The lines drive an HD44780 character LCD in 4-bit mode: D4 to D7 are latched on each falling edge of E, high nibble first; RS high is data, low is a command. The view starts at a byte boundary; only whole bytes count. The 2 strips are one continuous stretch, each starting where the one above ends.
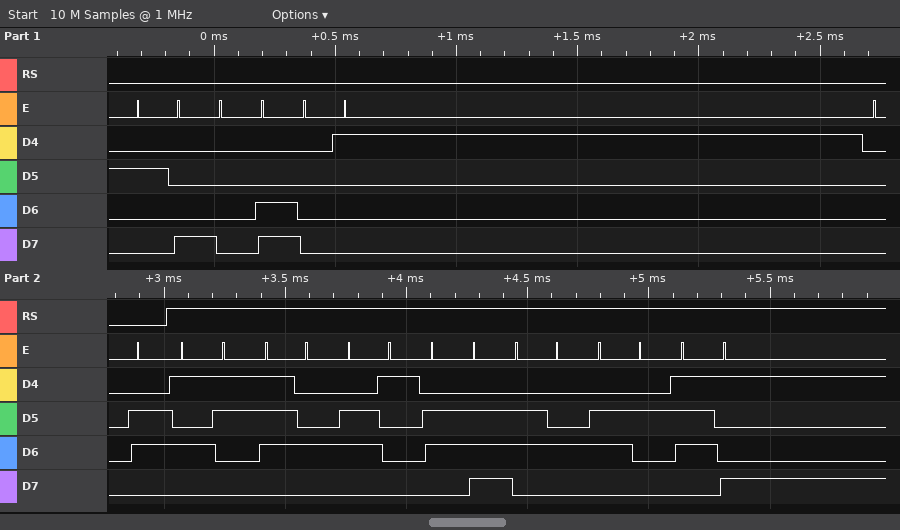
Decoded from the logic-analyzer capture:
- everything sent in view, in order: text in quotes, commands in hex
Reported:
0x28 0x0C 0x01 0x06 "Standby"
